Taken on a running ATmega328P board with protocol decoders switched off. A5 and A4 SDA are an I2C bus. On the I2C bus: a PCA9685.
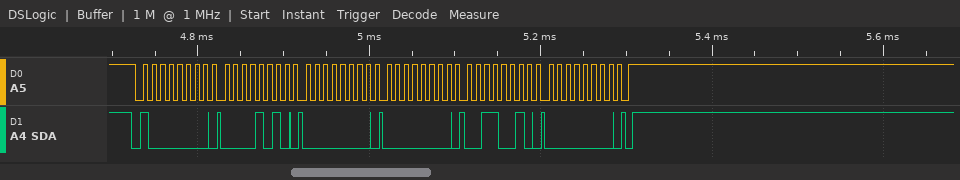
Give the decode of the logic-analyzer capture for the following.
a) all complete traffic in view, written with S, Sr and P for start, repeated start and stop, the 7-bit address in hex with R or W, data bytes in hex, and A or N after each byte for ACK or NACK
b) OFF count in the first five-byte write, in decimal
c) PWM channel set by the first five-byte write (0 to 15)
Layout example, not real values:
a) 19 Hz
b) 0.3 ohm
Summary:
a) S 40W A 0A A 00 A 00 A 32 A 00 A P
b) 50
c) 1
